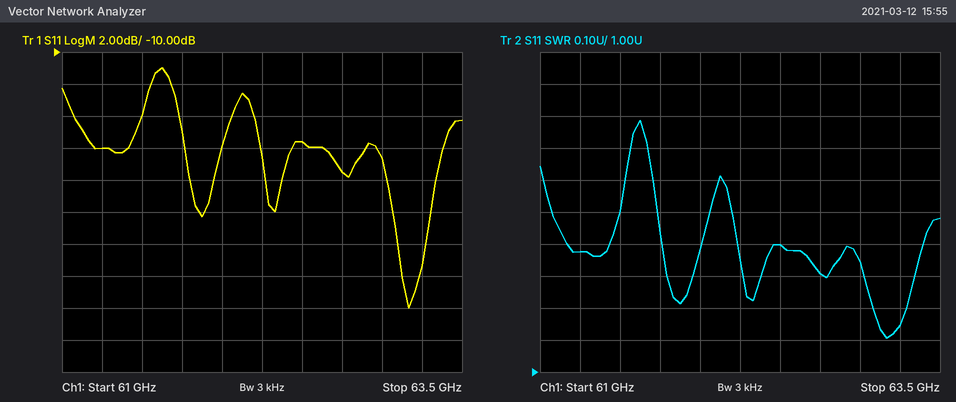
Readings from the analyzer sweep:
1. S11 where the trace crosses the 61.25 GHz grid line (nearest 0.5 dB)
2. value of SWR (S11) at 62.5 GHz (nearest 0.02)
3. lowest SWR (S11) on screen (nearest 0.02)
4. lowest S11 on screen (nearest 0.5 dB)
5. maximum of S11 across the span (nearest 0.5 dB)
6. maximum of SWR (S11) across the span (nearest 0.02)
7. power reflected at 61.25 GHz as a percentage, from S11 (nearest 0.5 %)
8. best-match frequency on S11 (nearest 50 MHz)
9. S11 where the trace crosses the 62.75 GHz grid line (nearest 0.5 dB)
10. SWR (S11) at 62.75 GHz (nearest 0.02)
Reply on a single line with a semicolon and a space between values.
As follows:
-16.0 dB; 1.40; 1.10; -26.0 dB; -11.0 dB; 1.78; 2.5 %; 63.15 GHz; -17.5 dB; 1.30
